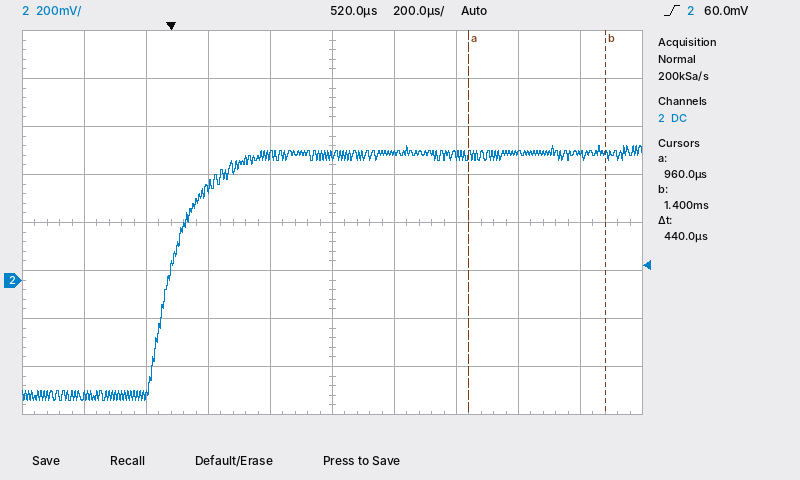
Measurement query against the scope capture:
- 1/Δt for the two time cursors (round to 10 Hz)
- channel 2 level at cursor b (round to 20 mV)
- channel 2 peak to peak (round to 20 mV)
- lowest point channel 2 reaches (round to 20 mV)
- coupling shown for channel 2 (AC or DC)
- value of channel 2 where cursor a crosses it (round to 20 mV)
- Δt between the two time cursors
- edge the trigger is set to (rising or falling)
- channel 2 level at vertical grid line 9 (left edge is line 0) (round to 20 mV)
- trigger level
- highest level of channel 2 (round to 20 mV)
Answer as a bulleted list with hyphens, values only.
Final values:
- 2.27 kHz
- 520 mV
- 1.06 V
- -500 mV
- DC
- 520 mV
- 440 µs
- rising
- 520 mV
- 60.0 mV
- 560 mV
